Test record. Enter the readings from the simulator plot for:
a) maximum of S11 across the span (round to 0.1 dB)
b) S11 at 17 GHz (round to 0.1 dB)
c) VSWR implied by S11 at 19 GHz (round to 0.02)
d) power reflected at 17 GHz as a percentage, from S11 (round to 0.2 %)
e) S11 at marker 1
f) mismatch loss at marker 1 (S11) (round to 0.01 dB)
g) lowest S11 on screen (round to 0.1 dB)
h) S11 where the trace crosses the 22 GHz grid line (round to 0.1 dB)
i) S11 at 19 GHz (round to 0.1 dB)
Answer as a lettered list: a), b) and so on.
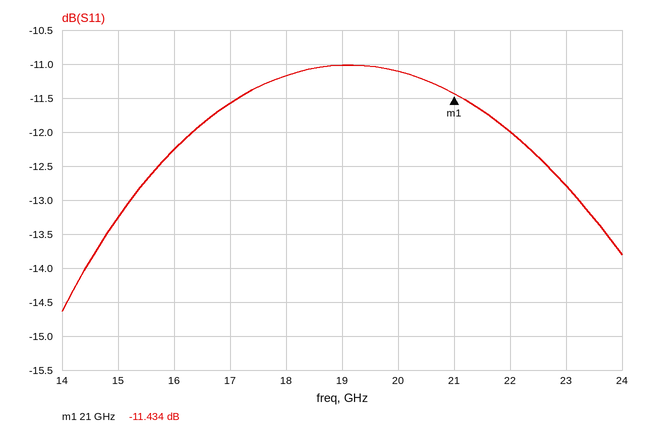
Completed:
a) -11.0 dB
b) -11.6 dB
c) 1.78
d) 7.0 %
e) -11.434 dB
f) 0.32 dB
g) -14.6 dB
h) -12.0 dB
i) -11.0 dB
